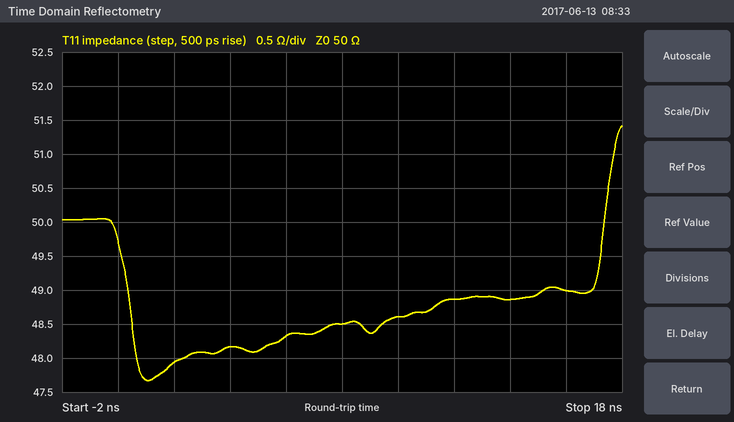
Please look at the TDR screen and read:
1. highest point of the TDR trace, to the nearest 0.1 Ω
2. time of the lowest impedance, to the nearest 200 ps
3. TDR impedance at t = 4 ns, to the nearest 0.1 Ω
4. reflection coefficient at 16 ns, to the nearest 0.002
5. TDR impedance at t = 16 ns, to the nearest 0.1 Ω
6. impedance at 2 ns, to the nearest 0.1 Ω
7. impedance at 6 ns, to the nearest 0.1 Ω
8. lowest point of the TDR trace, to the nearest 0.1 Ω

51.4 Ω
1.0 ns
48.2 Ω
-0.010
49.0 Ω
47.9 Ω
48.3 Ω
47.7 Ω
